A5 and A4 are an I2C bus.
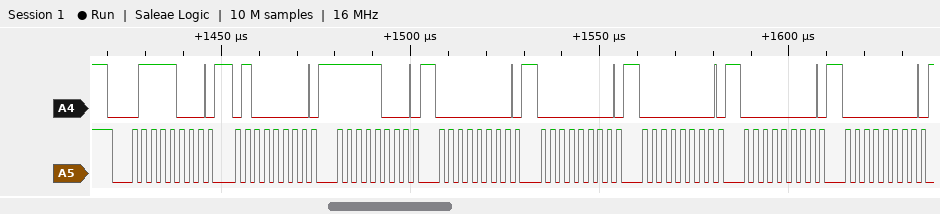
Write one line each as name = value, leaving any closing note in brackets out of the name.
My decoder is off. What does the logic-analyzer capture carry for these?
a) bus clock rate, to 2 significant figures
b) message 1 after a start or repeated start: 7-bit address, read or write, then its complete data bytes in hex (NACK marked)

bus clock rate, to 2 significant figures = 400 kHz
message 1 after a start or repeated start: 7-bit address, read or write, then its complete data bytes in hex = 0x3C write: 40 F8 00 00 00 00 00
